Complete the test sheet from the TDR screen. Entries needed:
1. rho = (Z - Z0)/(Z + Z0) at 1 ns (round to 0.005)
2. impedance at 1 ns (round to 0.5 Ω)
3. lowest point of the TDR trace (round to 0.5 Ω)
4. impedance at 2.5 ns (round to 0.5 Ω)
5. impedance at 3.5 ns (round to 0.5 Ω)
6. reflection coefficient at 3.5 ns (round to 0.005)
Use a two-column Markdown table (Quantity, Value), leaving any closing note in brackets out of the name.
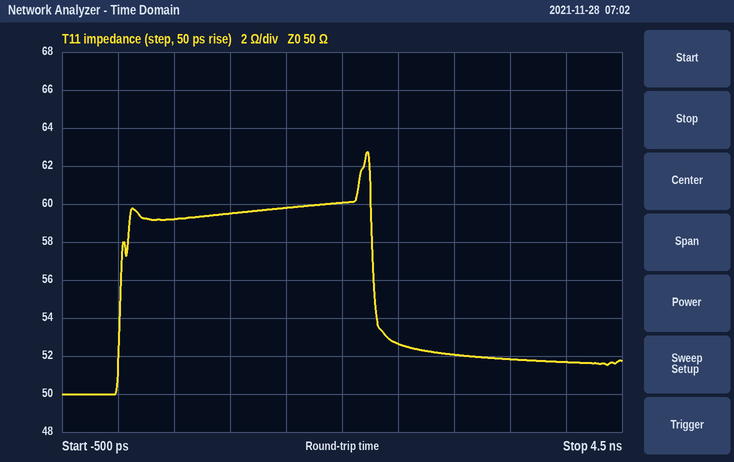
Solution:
| Quantity | Value |
|---|---|
| rho = (Z - Z0)/(Z + Z0) at 1 ns | +0.085 |
| impedance at 1 ns | 59.5 Ω |
| lowest point of the TDR trace | 50.0 Ω |
| impedance at 2.5 ns | 52.5 Ω |
| impedance at 3.5 ns | 52.0 Ω |
| reflection coefficient at 3.5 ns | +0.020 |
